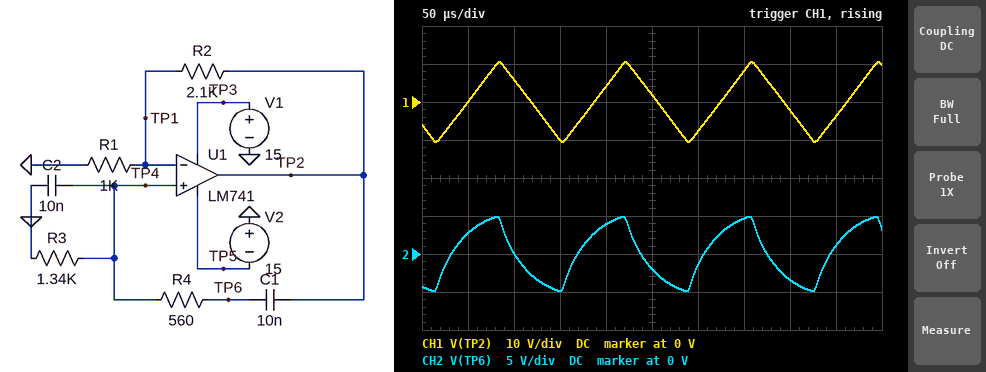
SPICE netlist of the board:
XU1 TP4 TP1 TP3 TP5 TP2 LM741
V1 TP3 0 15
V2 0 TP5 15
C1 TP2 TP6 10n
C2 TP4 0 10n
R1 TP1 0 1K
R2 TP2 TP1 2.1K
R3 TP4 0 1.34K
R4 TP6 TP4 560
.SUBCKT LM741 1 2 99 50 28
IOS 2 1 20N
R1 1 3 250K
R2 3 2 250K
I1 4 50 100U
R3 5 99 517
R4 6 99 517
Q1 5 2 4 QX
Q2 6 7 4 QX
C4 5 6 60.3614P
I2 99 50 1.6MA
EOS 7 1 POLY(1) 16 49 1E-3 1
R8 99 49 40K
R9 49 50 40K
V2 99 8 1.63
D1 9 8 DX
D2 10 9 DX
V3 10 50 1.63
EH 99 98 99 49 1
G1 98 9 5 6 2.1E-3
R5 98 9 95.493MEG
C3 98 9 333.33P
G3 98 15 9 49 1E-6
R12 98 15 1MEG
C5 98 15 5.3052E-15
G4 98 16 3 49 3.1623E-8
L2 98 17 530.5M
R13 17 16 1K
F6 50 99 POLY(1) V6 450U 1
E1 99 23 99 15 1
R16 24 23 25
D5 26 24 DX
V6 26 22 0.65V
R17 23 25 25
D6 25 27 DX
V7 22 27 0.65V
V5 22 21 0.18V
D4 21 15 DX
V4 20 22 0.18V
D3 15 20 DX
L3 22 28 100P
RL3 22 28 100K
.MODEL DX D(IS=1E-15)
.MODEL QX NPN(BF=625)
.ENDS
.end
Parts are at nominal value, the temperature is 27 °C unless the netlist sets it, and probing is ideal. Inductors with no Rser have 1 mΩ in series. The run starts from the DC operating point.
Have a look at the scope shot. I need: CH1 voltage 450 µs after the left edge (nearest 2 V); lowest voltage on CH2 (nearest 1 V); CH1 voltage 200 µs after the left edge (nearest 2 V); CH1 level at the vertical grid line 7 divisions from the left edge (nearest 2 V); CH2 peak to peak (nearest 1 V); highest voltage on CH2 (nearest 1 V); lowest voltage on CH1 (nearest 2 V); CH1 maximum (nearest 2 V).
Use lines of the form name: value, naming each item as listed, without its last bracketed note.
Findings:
CH1 voltage 450 µs after the left edge: -4 V
lowest voltage on CH2: -5 V
CH1 voltage 200 µs after the left edge: 4 V
CH1 level at the vertical grid line 7 divisions from the left edge: 8 V
CH2 peak to peak: 10 V
highest voltage on CH2: 5 V
lowest voltage on CH1: -10 V
CH1 maximum: 10 V
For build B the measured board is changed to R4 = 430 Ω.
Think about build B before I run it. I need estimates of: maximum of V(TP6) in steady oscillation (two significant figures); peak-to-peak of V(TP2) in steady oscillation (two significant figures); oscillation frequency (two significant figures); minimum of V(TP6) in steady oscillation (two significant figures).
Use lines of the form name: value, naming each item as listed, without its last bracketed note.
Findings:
maximum of V(TP6) in steady oscillation: 4.7 V
peak-to-peak of V(TP2) in steady oscillation: 22 V
oscillation frequency: 7.1 kHz
minimum of V(TP6) in steady oscillation: -4.7 V
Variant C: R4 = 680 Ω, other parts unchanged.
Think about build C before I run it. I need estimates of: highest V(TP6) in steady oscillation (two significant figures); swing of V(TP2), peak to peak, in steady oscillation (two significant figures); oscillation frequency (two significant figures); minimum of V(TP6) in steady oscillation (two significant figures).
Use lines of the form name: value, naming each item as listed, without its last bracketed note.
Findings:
highest V(TP6) in steady oscillation: 5.1 V
swing of V(TP2), peak to peak, in steady oscillation: 20 V
oscillation frequency: 7.5 kHz
minimum of V(TP6) in steady oscillation: -5.1 V
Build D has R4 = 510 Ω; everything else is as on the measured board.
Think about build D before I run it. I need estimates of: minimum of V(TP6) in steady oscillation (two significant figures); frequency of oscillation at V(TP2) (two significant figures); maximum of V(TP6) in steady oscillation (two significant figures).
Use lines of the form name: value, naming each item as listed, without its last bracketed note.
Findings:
minimum of V(TP6) in steady oscillation: -4.8 V
frequency of oscillation at V(TP2): 7.2 kHz
maximum of V(TP6) in steady oscillation: 4.8 V
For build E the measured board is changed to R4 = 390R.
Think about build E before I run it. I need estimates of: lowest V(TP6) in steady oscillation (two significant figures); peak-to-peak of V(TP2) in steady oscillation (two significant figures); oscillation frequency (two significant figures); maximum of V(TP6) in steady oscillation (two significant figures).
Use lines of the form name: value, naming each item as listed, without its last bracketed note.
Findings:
lowest V(TP6) in steady oscillation: -4.6 V
peak-to-peak of V(TP2) in steady oscillation: 22 V
oscillation frequency: 7.1 kHz
maximum of V(TP6) in steady oscillation: 4.6 V
